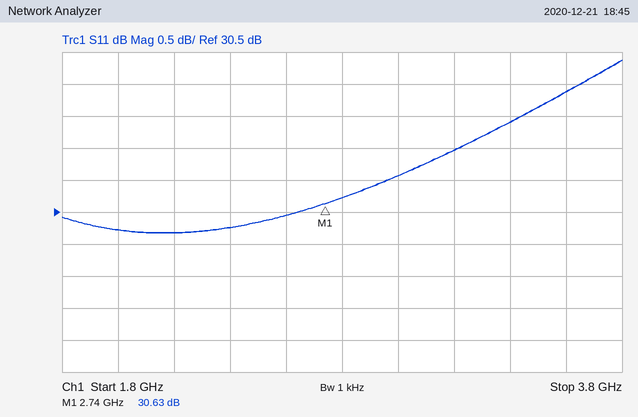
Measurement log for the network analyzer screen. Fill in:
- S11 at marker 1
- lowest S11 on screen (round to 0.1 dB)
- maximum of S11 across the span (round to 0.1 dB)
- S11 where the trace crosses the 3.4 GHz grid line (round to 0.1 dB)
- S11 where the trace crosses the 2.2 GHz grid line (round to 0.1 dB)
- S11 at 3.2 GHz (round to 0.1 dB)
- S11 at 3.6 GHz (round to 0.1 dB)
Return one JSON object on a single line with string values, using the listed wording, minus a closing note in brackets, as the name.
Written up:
{"S11 at marker 1": "30.63 dB", "lowest S11 on screen": "30.2 dB", "maximum of S11 across the span": "32.9 dB", "S11 where the trace crosses the 3.4 GHz grid line": "31.9 dB", "S11 where the trace crosses the 2.2 GHz grid line": "30.2 dB", "S11 at 3.2 GHz": "31.5 dB", "S11 at 3.6 GHz": "32.4 dB"}
